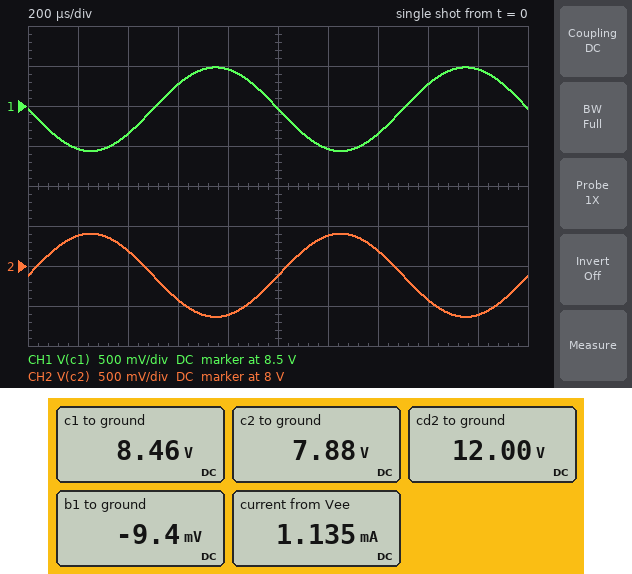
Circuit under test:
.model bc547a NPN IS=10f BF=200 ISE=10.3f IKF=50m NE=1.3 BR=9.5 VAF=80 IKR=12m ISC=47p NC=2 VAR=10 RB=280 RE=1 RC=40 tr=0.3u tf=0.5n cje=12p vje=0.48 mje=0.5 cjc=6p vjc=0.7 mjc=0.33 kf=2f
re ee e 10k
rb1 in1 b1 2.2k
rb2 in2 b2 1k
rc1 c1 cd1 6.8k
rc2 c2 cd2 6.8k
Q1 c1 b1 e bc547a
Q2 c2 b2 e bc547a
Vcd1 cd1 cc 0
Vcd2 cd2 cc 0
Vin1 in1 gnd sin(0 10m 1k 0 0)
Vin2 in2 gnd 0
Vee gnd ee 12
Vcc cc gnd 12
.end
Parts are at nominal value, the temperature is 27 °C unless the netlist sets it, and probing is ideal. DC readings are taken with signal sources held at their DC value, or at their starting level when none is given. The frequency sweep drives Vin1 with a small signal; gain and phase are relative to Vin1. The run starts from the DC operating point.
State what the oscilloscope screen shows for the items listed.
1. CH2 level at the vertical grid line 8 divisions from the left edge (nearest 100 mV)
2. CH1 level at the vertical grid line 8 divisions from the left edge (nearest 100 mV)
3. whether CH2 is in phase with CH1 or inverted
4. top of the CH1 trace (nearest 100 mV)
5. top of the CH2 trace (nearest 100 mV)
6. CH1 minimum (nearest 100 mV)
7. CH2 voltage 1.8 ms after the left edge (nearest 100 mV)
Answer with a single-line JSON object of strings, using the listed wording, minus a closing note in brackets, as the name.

{"CH2 level at the vertical grid line 8 divisions from the left edge": "7.6 V", "CH1 level at the vertical grid line 8 divisions from the left edge": "8.8 V", "whether CH2 is in phase with CH1 or inverted": "inverted", "top of the CH1 trace": "9.0 V", "top of the CH2 trace": "8.4 V", "CH1 minimum": "7.9 V", "CH2 voltage 1.8 ms after the left edge": "7.4 V"}
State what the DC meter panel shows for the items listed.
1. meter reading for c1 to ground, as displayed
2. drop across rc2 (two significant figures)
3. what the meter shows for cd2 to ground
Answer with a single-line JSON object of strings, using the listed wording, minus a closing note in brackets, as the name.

{"meter reading for c1 to ground, as displayed": "8.46 V", "drop across rc2": "4.1 V", "what the meter shows for cd2 to ground": "12.00 V"}
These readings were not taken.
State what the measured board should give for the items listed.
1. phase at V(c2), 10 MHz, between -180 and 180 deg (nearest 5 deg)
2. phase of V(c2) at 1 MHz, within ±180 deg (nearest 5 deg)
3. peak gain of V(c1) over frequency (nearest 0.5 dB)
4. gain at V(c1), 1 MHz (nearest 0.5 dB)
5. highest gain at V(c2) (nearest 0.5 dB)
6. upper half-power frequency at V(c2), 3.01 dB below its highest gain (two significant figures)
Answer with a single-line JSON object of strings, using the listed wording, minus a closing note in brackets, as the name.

{"phase at V(c2), 10 MHz, between -180 and 180 deg": "-90 deg", "phase of V(c2) at 1 MHz, within ±180 deg": "-75 deg", "peak gain of V(c1) over frequency": "34.5 dB", "gain at V(c1), 1 MHz": "22.5 dB", "highest gain at V(c2)": "34.5 dB", "upper half-power frequency at V(c2), 3.01 dB below its highest gain": "270 kHz"}
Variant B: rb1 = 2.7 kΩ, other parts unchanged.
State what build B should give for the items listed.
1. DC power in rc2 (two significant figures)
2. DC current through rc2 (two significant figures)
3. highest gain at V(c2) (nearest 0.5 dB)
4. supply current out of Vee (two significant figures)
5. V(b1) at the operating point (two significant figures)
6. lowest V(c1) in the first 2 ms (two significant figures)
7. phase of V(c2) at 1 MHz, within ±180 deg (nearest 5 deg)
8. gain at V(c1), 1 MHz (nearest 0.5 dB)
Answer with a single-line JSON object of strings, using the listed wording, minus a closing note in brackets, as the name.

{"DC power in rc2": "2.6 mW", "DC current through rc2": "620 µA", "highest gain at V(c2)": "34.0 dB", "supply current out of Vee": "1.1 mA", "V(b1) at the operating point": "-11 mV", "lowest V(c1) in the first 2 ms": "8.1 V", "phase of V(c2) at 1 MHz, within ±180 deg": "-80 deg", "gain at V(c1), 1 MHz": "21.5 dB"}
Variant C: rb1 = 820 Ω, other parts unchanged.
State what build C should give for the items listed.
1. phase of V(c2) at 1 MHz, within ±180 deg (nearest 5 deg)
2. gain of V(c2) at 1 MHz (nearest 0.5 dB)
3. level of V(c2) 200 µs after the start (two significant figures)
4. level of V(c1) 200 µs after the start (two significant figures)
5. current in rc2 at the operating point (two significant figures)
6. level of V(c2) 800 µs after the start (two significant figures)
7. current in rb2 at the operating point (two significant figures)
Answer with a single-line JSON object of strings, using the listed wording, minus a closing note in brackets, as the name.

{"phase of V(c2) at 1 MHz, within ±180 deg": "-70 deg", "gain of V(c2) at 1 MHz": "26.0 dB", "level of V(c2) 200 µs after the start": "8.8 V", "level of V(c1) 200 µs after the start": "7.6 V", "current in rc2 at the operating point": "560 µA", "level of V(c2) 800 µs after the start": "7.7 V", "current in rb2 at the operating point": "4.6 µA"}
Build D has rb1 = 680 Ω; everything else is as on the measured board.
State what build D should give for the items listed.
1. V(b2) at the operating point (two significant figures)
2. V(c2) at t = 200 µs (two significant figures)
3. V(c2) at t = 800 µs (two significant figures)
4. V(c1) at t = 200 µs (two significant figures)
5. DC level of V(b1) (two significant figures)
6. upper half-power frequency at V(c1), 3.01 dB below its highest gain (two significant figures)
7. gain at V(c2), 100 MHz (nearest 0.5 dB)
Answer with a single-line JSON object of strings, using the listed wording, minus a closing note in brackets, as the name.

{"V(b2) at the operating point": "-4.5 mV", "V(c2) at t = 200 µs": "8.8 V", "V(c2) at t = 800 µs": "7.7 V", "V(c1) at t = 200 µs": "7.5 V", "DC level of V(b1)": "-3.2 mV", "upper half-power frequency at V(c1), 3.01 dB below its highest gain": "400 kHz", "gain at V(c2), 100 MHz": "-9.0 dB"}
